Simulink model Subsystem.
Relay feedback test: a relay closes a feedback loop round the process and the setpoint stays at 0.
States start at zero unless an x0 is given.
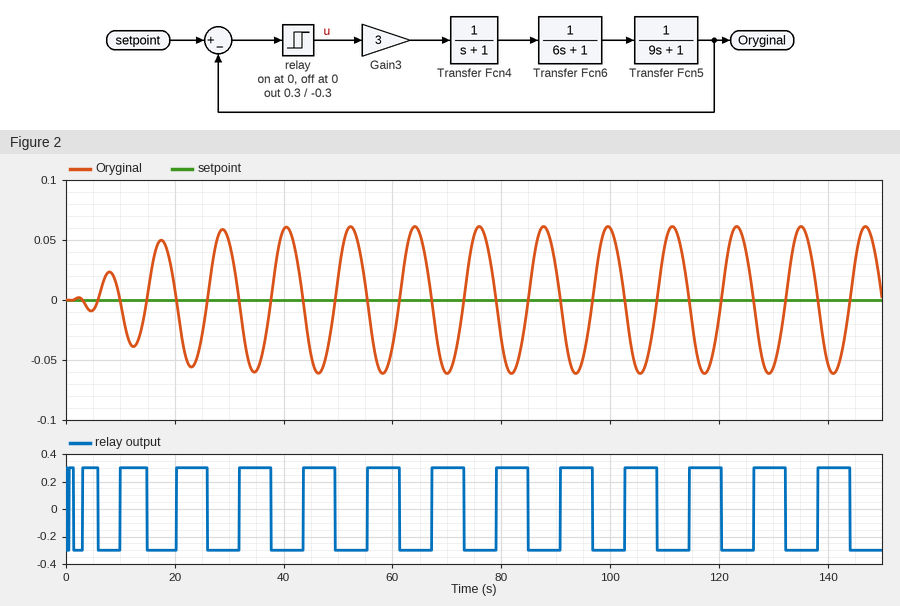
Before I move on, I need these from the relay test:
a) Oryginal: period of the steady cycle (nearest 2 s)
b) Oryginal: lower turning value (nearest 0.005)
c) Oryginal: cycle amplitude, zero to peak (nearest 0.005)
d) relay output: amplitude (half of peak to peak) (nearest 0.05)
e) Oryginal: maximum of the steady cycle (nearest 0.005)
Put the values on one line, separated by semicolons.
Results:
12 s; -0.060; 0.060; 0.30; 0.060
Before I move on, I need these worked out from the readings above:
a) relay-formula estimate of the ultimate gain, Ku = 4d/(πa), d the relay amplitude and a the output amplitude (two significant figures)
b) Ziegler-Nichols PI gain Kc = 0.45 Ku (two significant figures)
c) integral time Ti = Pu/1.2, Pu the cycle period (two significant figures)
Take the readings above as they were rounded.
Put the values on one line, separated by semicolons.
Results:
6.4; 2.9; 10 s
